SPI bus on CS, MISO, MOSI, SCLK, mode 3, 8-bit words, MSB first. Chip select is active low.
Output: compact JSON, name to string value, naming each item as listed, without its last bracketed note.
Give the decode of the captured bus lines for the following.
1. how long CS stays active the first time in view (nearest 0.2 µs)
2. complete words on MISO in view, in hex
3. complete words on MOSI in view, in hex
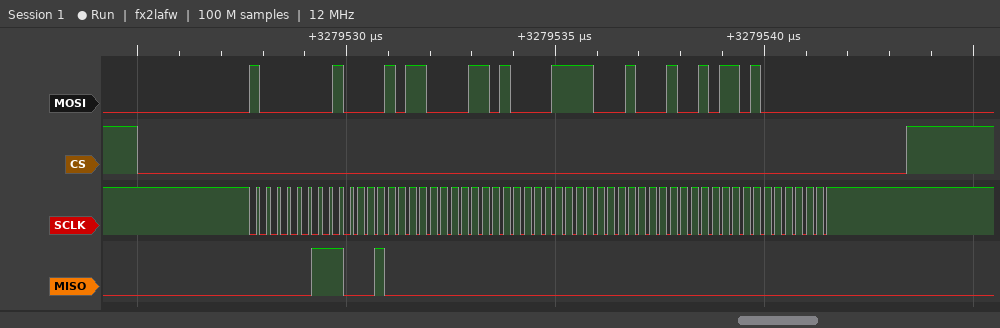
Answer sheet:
{"how long CS stays active the first time in view": "18.4 µs", "complete words on MISO in view, in hex": "03, 88, 00, 00, 00, 00, 00", "complete words on MOSI in view, in hex": "80, 85, 86, 87, 88, 96, 80"}
